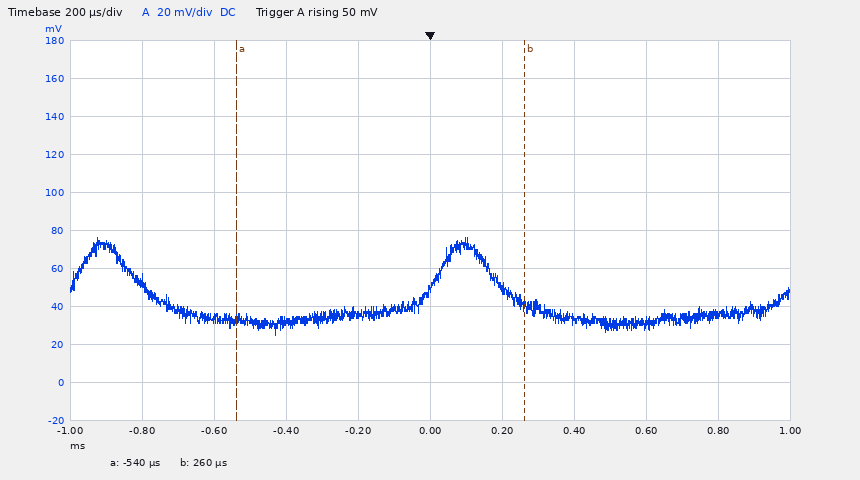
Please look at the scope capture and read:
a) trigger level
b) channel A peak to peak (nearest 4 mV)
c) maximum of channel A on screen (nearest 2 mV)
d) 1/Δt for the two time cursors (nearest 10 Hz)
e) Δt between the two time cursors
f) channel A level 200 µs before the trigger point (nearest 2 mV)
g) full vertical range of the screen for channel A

50 mV
52 mV
76 mV
1.25 kHz
800 µs
36 mV
200 mV
